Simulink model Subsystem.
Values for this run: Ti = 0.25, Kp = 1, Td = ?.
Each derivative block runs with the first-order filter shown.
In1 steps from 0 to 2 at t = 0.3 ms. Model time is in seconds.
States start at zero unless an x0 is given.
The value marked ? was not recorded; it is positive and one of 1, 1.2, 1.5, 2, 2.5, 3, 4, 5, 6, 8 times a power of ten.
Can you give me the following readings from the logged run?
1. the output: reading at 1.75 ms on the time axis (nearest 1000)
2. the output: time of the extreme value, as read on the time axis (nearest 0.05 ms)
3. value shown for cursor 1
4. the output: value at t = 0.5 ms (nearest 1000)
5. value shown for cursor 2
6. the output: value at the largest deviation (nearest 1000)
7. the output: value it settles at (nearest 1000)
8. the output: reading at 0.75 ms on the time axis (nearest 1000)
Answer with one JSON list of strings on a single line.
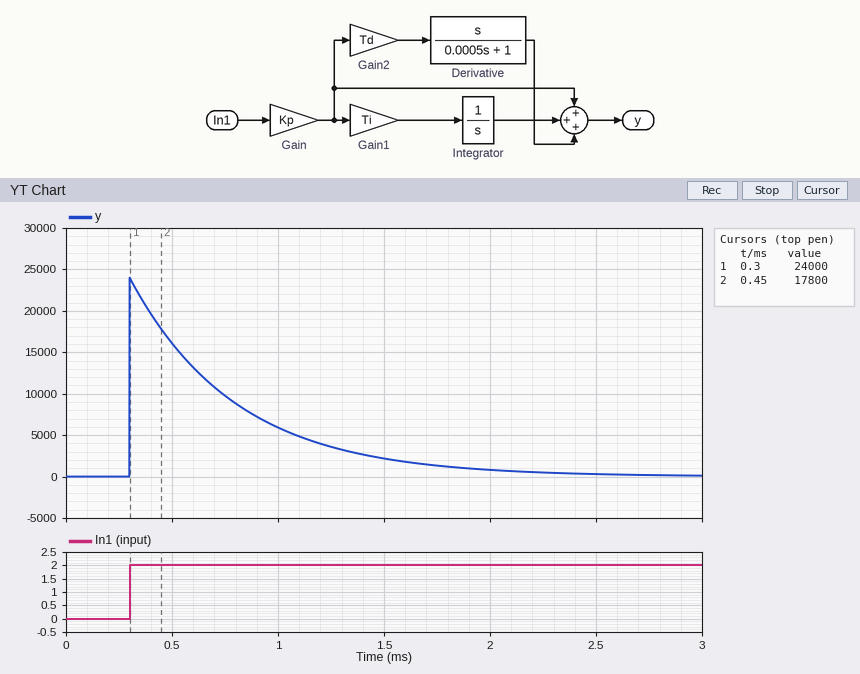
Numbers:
["1000", "0.30 ms", "24000", "16000", "17800", "24000", "0", "10000"]
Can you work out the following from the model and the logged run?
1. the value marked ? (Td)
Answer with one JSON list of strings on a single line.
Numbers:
["6"]
